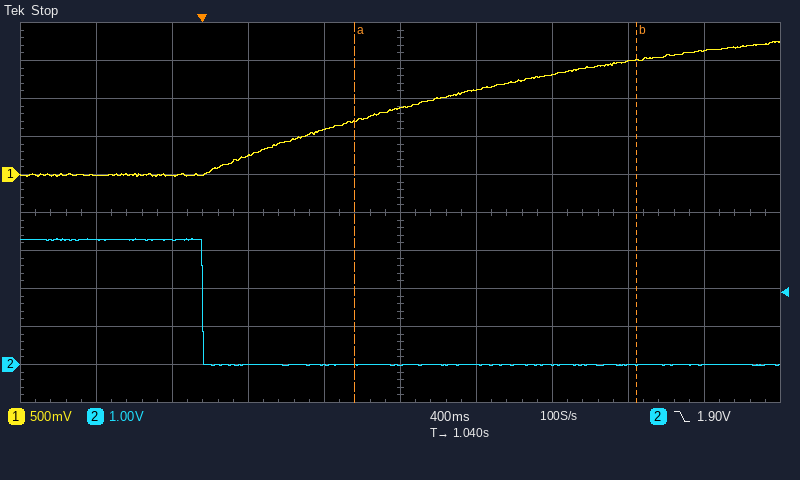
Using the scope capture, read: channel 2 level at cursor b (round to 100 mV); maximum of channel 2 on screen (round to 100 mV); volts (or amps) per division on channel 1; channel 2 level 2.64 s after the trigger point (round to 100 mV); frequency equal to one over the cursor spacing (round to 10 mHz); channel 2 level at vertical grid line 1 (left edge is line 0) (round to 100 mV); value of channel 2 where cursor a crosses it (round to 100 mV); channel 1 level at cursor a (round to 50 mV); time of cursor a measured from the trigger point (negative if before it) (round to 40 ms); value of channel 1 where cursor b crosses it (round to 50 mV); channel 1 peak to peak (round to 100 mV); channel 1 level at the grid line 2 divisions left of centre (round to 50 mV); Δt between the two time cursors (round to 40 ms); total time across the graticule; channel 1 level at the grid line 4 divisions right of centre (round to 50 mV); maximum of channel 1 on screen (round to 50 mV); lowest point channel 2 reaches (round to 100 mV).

0.0 V
3.3 V
500 mV
0.0 V
680 mHz
3.3 V
0.0 V
700 mV
+800 ms
1.50 V
1.80 V
250 mV
1.48 s
4 s
1.65 V
1.75 V
0.0 V
